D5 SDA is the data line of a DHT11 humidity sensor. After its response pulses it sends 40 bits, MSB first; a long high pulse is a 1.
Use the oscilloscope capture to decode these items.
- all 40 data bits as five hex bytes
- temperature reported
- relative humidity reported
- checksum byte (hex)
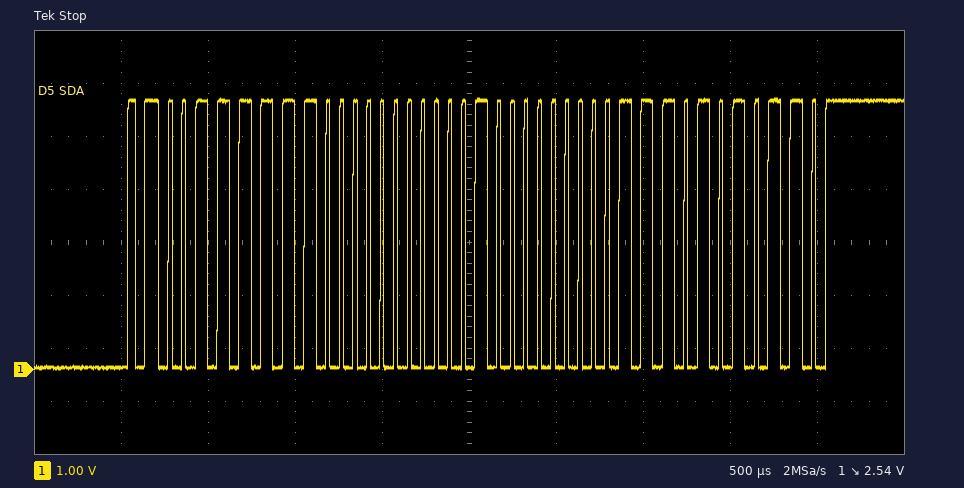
3F 00 10 07 56
16.7 °C
63 %
0x56
